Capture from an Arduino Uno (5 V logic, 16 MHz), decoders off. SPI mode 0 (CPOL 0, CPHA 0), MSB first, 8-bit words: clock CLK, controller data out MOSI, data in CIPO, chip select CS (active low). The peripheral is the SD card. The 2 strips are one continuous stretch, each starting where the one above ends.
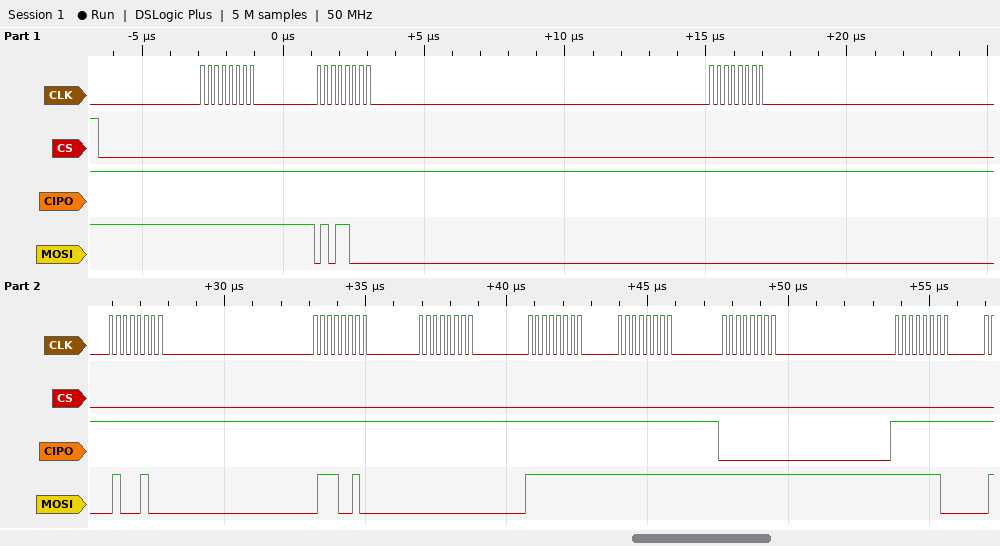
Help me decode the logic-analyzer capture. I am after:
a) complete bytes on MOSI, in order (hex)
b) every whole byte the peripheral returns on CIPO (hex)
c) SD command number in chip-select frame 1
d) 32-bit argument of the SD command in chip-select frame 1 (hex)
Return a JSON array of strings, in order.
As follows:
["FF 58 00 44 72 00 FF FF FF FE", "FF FF FF FF FF FF FF FF 00 FF", "CMD24", "0x00447200"]
